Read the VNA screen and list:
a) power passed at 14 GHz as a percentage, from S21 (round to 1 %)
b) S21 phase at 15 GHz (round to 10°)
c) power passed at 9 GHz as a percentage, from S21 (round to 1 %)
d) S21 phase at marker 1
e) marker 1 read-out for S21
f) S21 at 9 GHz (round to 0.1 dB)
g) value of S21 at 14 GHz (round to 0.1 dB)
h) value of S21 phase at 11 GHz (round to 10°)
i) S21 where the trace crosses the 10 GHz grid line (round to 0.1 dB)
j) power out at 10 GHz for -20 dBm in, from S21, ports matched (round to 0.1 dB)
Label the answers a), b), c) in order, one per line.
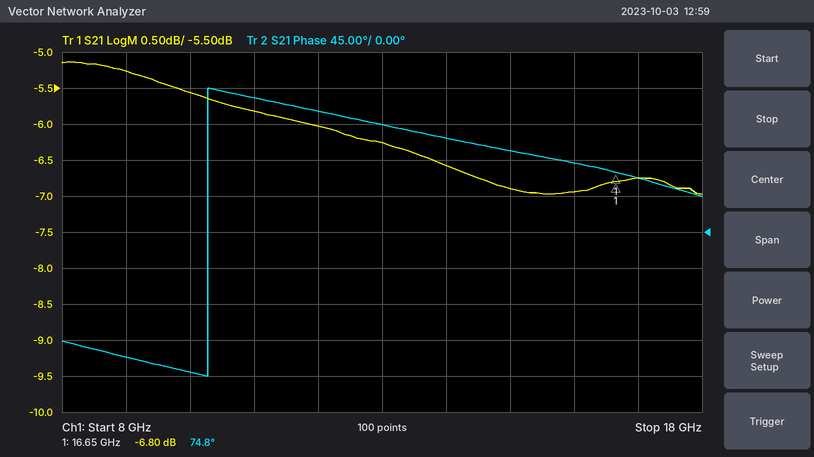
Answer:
a) 22 %
b) 100°
c) 30 %
d) 74.8°
e) -6.80 dB
f) -5.3 dB
g) -6.6 dB
h) 170°
i) -5.6 dB
j) -25.6 dBm
